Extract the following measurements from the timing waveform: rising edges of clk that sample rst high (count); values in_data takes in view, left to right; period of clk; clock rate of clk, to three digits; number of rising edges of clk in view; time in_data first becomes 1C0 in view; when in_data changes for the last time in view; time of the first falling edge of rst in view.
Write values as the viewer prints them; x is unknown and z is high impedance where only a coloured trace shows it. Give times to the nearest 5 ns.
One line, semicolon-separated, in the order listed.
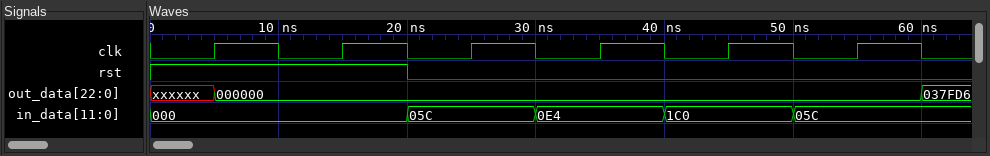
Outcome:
2; 000, 05C, 0E4, 1C0, 05C; 10 ns; 100 MHz; 6; 40 ns; 50 ns; 20 ns
